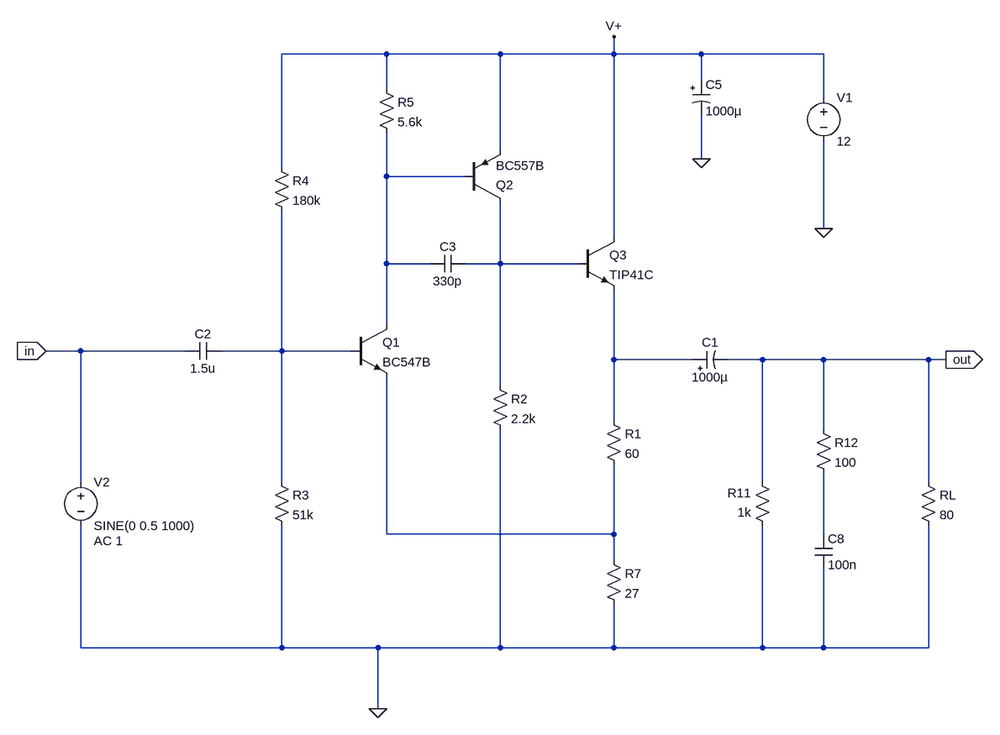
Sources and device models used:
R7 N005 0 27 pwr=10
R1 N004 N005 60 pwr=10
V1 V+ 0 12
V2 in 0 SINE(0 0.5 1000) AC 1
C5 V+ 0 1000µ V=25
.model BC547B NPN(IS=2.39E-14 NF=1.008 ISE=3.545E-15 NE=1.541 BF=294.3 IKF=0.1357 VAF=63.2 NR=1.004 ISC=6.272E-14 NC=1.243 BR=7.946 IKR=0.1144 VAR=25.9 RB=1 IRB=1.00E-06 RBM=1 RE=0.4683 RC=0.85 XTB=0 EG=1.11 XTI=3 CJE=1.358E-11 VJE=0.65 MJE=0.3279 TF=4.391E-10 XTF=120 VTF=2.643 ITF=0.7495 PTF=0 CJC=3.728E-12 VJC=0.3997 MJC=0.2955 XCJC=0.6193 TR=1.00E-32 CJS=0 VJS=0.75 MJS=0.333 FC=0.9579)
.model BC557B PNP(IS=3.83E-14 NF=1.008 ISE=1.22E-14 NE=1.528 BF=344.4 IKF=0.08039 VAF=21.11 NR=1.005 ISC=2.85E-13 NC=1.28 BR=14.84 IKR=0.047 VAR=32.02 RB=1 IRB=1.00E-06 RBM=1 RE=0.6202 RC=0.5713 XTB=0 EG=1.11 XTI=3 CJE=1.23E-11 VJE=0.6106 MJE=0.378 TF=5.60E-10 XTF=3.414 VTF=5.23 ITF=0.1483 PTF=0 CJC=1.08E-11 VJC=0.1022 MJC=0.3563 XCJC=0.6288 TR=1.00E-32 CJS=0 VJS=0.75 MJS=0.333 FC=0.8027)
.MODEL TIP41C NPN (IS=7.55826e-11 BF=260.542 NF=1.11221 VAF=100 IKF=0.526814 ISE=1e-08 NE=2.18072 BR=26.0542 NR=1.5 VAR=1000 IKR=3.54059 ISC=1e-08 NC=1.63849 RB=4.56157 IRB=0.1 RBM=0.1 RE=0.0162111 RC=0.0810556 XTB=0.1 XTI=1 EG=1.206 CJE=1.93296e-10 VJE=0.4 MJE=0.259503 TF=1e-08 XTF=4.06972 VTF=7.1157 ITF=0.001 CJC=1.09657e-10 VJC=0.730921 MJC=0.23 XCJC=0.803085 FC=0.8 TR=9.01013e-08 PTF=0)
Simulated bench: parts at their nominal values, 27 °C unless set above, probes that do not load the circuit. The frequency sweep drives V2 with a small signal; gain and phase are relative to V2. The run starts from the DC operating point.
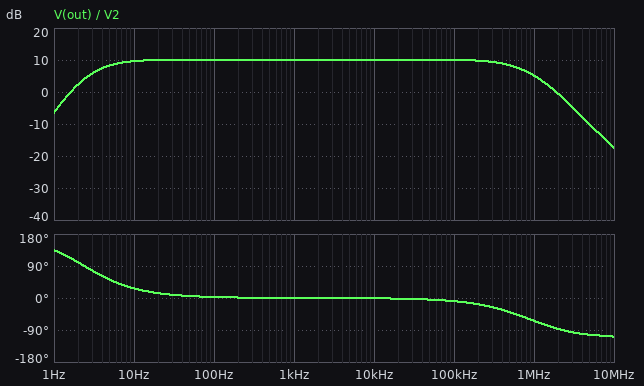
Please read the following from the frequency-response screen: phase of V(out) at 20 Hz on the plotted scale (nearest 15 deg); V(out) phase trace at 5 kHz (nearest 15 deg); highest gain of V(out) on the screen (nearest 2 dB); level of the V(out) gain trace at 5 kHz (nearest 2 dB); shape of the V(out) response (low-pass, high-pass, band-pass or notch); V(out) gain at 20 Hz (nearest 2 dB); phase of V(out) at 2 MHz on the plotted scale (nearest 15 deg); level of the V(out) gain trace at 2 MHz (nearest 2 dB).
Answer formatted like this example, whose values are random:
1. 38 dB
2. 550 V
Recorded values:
1. 15 deg
2. 0 deg
3. 10 dB
4. 10 dB
5. band-pass
6. 10 dB
7. -90 deg
8. 0 dB
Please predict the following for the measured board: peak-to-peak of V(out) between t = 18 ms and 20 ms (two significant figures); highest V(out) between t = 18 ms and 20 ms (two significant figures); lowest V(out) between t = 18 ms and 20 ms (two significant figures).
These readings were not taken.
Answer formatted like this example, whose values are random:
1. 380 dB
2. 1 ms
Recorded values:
1. 3.2 V
2. 1.6 V
3. -1.6 V
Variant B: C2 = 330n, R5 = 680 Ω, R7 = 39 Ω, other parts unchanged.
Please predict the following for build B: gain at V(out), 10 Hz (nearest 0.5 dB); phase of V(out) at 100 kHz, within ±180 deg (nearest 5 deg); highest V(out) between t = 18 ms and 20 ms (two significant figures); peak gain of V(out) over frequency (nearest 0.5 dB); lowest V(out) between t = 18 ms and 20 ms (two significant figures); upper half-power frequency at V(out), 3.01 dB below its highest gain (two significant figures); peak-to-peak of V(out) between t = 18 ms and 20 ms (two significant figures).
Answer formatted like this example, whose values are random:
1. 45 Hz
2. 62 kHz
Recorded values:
1. 4.0 dB
2. 0 deg
3. 1.3 V
4. 8.0 dB
5. -1.3 V
6. 3.6 MHz
7. 2.5 V
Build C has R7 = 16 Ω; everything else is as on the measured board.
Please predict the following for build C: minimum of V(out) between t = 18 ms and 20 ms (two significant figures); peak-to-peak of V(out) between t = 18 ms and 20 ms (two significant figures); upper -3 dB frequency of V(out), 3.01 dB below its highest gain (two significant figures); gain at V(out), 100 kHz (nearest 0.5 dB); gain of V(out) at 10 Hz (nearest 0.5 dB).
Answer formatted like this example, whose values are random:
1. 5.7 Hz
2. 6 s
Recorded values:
1. -2.4 V
2. 4.1 V
3. 510 kHz
4. 13.5 dB
5. 13.0 dB
